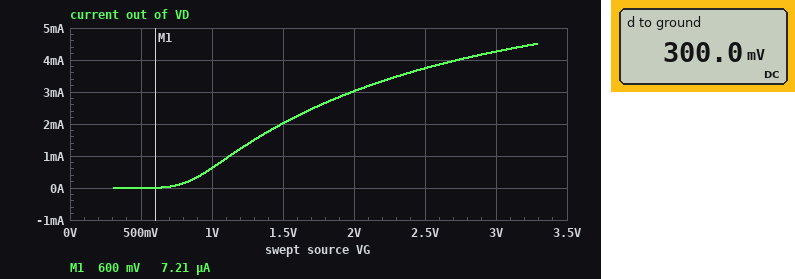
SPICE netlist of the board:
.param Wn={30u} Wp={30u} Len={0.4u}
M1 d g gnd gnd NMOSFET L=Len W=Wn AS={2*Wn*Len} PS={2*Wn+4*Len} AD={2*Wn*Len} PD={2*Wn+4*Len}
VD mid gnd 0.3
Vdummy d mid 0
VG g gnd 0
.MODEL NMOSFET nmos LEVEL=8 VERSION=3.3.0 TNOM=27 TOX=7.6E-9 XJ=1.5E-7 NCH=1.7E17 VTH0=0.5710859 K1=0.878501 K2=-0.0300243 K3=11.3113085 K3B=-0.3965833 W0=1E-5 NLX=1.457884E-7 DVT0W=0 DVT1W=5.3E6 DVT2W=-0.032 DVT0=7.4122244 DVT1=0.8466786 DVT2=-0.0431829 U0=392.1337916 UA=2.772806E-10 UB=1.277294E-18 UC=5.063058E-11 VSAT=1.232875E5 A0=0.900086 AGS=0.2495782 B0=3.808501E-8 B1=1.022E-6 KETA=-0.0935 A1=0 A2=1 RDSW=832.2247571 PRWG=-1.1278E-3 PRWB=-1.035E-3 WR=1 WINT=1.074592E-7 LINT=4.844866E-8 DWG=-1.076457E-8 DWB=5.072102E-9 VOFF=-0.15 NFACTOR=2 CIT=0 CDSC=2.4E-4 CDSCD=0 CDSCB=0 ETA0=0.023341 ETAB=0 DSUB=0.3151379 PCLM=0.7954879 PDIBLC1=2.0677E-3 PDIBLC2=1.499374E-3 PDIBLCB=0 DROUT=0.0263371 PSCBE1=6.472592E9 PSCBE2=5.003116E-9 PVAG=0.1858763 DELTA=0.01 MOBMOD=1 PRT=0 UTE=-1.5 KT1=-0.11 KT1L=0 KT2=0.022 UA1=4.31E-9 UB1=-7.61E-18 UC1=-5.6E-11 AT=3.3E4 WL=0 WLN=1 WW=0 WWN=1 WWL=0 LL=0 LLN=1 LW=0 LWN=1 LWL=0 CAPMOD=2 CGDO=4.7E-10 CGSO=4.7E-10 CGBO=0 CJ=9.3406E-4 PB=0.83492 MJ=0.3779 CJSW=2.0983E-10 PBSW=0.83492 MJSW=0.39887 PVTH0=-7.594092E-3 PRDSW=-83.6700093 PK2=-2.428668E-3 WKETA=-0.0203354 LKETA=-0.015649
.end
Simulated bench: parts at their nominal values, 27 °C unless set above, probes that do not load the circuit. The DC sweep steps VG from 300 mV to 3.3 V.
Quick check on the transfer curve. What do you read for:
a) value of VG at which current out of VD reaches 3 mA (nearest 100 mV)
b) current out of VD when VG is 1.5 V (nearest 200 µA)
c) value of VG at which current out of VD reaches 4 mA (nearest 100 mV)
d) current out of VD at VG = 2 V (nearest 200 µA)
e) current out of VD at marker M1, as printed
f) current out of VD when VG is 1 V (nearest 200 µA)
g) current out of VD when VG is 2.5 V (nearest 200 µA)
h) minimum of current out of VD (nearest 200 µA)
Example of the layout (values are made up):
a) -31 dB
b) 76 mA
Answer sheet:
a) 2.0 V
b) 2.0 mA
c) 2.7 V
d) 3.0 mA
e) 7.21 µA
f) 600 µA
g) 3.8 mA
h) 0 A
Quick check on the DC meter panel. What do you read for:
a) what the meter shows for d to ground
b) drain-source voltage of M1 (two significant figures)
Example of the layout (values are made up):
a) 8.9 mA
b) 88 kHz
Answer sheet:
a) 300.0 mV
b) 300 mV
